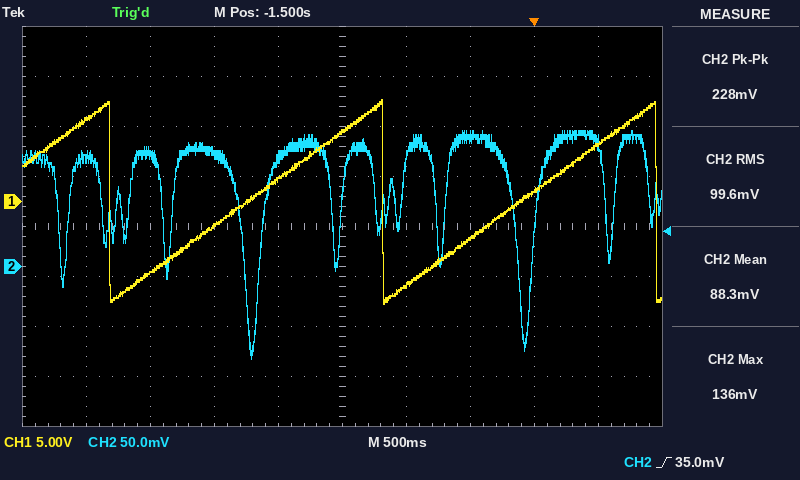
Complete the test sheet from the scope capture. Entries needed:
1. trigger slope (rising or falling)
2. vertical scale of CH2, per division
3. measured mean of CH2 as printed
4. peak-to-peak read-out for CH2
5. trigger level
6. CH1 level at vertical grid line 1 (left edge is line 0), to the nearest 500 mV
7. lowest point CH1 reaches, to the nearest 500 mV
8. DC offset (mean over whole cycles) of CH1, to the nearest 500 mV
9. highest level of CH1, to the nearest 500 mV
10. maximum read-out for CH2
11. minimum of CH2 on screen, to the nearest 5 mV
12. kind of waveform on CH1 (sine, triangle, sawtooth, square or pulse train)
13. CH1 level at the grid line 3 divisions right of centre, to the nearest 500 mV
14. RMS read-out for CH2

rising
50 mV
88.3 mV
228 mV
35.0 mV
8.0 V
-10.0 V
0.0 V
10.0 V
136 mV
-90 mV
sawtooth
1.0 V
99.6 mV
